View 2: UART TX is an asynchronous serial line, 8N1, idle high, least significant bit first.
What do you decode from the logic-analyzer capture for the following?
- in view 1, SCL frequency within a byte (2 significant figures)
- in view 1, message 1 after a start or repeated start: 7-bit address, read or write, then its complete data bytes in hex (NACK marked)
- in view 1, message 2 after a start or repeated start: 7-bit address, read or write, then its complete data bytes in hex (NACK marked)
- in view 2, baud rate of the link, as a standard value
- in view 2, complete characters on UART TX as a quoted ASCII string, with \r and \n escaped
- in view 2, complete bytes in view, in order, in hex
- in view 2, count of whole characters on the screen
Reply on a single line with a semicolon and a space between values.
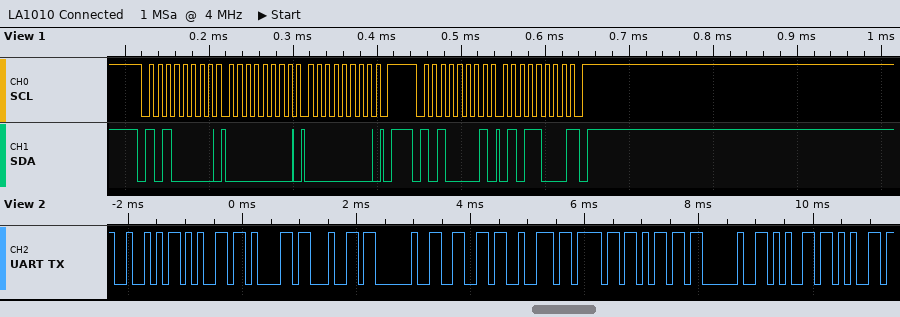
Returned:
100 kHz; 0x50 write: 00 00; 0x50 read: 58 NACK; 9600 baud; "Read from ee"; 52 65 61 64 20 66 72 6F 6D 20 65 65; 12
